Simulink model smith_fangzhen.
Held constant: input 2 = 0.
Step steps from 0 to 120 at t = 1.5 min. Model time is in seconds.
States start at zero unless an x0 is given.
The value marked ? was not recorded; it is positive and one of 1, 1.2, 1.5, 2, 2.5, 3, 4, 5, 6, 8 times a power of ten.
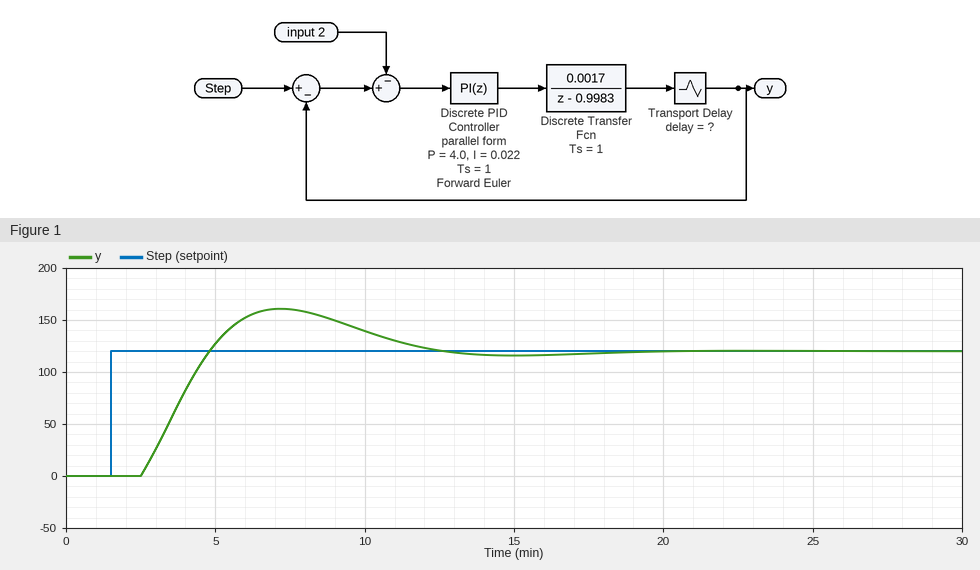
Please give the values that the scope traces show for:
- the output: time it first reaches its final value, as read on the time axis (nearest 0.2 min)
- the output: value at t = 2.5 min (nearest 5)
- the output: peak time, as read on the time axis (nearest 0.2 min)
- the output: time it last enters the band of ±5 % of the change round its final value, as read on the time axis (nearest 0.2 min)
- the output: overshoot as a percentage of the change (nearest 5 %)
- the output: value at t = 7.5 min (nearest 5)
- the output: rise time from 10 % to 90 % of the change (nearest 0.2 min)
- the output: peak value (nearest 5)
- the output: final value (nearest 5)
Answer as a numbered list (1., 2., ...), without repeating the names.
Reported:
1. 4.8 min
2. 0
3. 7.2 min
4. 11.6 min
5. 35 %
6. 160
7. 1.8 min
8. 160
9. 120
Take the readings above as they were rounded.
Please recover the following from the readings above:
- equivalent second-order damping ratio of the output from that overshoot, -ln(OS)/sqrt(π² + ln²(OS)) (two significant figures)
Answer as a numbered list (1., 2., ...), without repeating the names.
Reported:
1. 0.32
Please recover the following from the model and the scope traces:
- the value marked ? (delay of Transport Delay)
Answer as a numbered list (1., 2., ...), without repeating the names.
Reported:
1. 60
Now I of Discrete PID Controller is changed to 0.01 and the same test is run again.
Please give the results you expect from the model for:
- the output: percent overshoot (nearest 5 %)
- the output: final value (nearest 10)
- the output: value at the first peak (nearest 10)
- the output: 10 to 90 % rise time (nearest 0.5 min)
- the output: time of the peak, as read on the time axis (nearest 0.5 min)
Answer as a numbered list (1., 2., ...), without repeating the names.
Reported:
1. 10 %
2. 120
3. 130
4. 2.5 min
5. 8.0 min
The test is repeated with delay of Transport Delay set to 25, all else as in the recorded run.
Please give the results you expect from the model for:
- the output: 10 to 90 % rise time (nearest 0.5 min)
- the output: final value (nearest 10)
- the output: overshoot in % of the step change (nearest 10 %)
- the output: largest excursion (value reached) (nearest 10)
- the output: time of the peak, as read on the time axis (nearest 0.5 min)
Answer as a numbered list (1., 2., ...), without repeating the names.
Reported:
1. 2.5 min
2. 120
3. 20 %
4. 140
5. 8.0 min
